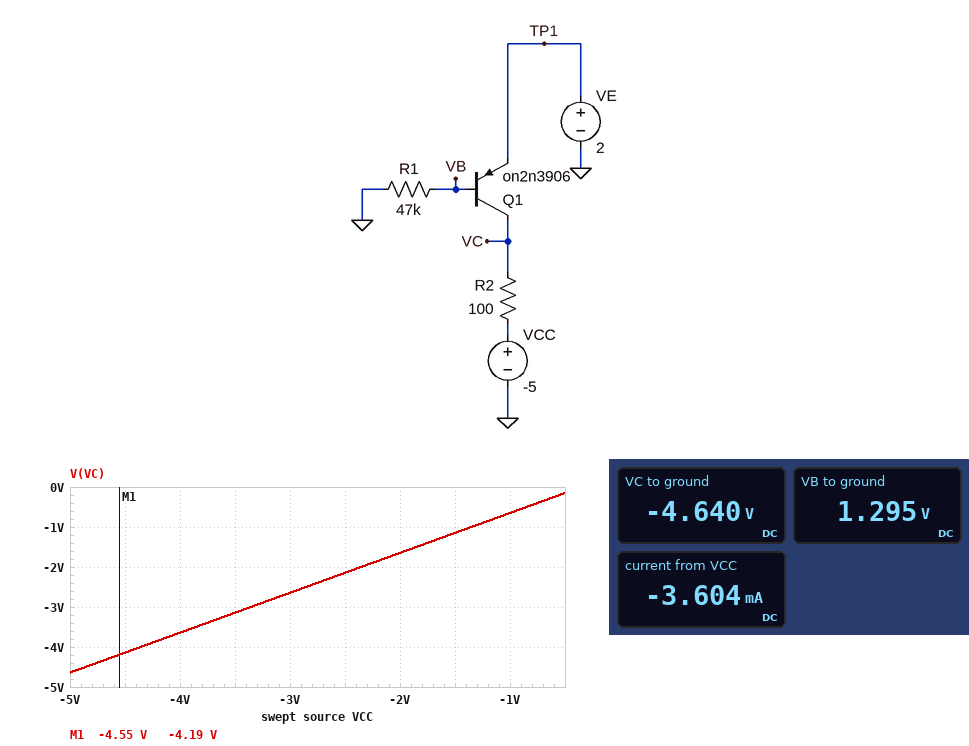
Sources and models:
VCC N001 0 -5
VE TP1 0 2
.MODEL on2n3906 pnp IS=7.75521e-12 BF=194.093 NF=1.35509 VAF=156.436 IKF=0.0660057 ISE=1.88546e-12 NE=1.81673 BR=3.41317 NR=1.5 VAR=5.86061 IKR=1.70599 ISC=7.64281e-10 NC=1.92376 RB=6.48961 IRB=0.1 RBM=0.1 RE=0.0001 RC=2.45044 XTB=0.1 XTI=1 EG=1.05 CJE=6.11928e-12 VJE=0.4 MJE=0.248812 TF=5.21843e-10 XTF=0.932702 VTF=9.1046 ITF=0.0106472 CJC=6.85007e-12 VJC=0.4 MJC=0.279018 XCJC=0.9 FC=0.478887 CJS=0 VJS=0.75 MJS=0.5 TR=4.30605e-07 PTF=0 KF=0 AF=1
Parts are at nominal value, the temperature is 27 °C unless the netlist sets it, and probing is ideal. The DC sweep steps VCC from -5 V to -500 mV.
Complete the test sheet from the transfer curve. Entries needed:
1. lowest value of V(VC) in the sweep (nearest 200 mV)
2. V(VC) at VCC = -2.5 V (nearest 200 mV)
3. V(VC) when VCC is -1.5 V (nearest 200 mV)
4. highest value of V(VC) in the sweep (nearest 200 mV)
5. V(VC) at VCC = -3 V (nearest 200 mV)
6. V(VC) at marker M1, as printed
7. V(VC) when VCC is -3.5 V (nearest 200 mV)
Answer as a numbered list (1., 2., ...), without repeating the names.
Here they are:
1. -4.6 V
2. -2.2 V
3. -1.2 V
4. -200 mV
5. -2.6 V
6. -4.19 V
7. -3.2 V
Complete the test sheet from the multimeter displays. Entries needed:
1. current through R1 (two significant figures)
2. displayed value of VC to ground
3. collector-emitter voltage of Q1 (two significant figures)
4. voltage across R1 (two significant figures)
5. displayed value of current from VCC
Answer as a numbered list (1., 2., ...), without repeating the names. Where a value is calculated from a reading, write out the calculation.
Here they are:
1. (1.295 V) / 47 kΩ = 28 µA
2. -4.640 V
3. -4.64 V - 2 V = -6.6 V
4. 1.295 V = 1.3 V
5. -3.604 mA
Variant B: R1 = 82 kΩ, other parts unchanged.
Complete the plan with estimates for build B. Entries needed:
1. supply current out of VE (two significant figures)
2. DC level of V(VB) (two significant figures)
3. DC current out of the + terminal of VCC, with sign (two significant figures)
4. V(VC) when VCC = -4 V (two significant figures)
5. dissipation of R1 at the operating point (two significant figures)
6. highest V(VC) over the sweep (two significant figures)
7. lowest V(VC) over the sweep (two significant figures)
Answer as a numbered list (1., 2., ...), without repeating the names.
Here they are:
1. 2.1 mA
2. 1.3 V
3. -2.1 mA
4. -3.8 V
5. 21 µW
6. -300 mV
7. -4.8 V
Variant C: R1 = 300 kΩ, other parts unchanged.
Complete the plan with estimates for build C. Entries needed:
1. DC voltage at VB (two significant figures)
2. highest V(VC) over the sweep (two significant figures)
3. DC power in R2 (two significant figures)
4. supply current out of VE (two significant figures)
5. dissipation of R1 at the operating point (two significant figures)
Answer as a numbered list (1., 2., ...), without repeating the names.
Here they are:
1. 1.4 V
2. -450 mV
3. 31 µW
4. 560 µA
5. 6.2 µW
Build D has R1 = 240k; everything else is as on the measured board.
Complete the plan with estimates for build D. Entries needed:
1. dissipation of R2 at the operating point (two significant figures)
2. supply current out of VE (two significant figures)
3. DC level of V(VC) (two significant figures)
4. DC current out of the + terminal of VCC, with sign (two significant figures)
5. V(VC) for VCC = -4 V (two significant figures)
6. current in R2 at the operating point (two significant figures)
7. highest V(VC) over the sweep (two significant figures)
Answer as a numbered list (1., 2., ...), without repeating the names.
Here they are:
1. 49 µW
2. 710 µA
3. -4.9 V
4. -700 µA
5. -3.9 V
6. 700 µA
7. -430 mV
